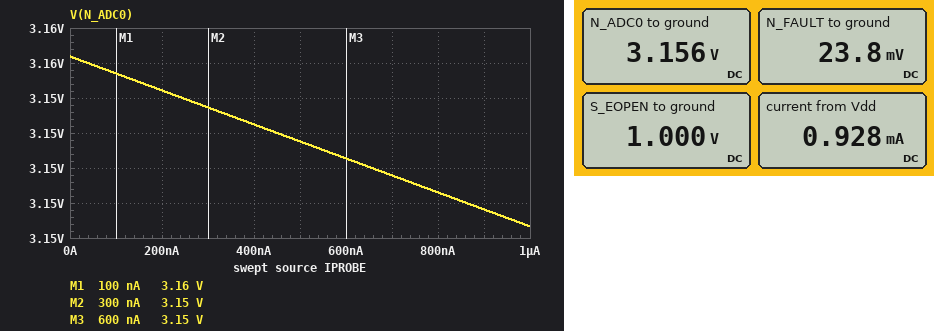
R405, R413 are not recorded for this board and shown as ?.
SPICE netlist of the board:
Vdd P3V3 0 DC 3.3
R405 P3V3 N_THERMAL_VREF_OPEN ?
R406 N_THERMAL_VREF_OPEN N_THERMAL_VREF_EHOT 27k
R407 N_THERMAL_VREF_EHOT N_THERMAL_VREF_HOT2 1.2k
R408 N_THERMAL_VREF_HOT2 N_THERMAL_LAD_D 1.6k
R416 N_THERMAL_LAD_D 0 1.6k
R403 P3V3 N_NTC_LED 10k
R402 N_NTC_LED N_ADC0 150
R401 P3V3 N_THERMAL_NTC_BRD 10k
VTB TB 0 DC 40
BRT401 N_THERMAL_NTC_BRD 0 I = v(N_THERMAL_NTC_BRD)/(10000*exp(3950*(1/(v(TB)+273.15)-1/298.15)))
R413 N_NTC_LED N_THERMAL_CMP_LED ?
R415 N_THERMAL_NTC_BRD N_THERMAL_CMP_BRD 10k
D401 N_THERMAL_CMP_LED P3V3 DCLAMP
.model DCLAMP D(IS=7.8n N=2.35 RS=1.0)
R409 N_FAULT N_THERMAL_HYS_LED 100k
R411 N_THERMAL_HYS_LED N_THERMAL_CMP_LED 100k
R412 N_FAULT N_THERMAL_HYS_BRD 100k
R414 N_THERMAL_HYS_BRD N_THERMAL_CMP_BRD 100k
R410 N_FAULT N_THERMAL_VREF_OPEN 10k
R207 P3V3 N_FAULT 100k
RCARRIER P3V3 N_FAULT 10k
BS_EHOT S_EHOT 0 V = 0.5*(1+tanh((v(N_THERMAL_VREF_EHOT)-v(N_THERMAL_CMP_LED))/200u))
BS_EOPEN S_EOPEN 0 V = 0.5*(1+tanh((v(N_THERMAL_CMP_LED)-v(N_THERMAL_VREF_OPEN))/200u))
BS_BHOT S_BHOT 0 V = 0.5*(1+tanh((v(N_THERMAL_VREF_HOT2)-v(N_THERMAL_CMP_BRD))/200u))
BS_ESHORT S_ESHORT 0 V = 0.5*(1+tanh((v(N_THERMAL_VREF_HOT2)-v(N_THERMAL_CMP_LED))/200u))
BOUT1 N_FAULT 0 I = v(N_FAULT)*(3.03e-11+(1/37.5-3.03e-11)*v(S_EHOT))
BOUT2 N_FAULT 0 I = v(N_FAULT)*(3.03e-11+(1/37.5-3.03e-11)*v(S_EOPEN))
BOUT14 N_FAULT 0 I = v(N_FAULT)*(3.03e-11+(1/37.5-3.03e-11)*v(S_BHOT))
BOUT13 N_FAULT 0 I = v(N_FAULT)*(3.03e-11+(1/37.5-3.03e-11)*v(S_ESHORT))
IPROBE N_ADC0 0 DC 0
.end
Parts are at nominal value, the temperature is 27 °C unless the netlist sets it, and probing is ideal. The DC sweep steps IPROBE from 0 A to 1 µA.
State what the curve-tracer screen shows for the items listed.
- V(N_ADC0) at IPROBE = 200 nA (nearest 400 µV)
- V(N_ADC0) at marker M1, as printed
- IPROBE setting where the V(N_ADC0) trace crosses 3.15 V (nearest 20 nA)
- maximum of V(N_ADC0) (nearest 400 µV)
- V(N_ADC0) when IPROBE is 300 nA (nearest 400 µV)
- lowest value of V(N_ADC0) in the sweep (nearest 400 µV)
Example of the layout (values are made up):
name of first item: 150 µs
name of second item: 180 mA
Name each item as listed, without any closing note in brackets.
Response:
V(N_ADC0) at IPROBE = 200 nA: 3.1544 V
V(N_ADC0) at marker M1, as printed: 3.16 V
IPROBE setting where the V(N_ADC0) trace crosses 3.15 V: 660 nA
maximum of V(N_ADC0): 3.1564 V
V(N_ADC0) when IPROBE is 300 nA: 3.1536 V
lowest value of V(N_ADC0) in the sweep: 3.1468 V
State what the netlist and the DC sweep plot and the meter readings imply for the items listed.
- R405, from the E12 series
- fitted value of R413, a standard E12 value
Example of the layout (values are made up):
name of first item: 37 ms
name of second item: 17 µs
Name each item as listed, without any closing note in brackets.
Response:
R405, from the E12 series: 2.2 kΩ
fitted value of R413, a standard E12 value: 18 kΩ
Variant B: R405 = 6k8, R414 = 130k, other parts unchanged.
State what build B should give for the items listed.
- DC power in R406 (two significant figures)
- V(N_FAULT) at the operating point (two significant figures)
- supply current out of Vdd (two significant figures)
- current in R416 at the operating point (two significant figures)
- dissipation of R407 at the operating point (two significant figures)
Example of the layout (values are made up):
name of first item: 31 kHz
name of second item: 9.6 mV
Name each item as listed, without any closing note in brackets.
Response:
DC power in R406: 84 µW
V(N_FAULT) at the operating point: 21 mV
supply current out of Vdd: 820 µA
current in R416 at the operating point: 56 µA
dissipation of R407 at the operating point: 3.7 µW
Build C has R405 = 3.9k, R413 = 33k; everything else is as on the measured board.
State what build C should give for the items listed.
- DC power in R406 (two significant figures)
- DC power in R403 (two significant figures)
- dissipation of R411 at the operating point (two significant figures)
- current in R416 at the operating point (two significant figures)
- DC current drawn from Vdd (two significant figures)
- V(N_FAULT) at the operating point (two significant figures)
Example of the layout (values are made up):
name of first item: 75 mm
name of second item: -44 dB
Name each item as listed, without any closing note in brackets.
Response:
DC power in R406: 130 µW
DC power in R403: 1.8 µW
dissipation of R411 at the operating point: 18 µW
current in R416 at the operating point: 70 µA
DC current drawn from Vdd: 880 µA
V(N_FAULT) at the operating point: 22 mV
